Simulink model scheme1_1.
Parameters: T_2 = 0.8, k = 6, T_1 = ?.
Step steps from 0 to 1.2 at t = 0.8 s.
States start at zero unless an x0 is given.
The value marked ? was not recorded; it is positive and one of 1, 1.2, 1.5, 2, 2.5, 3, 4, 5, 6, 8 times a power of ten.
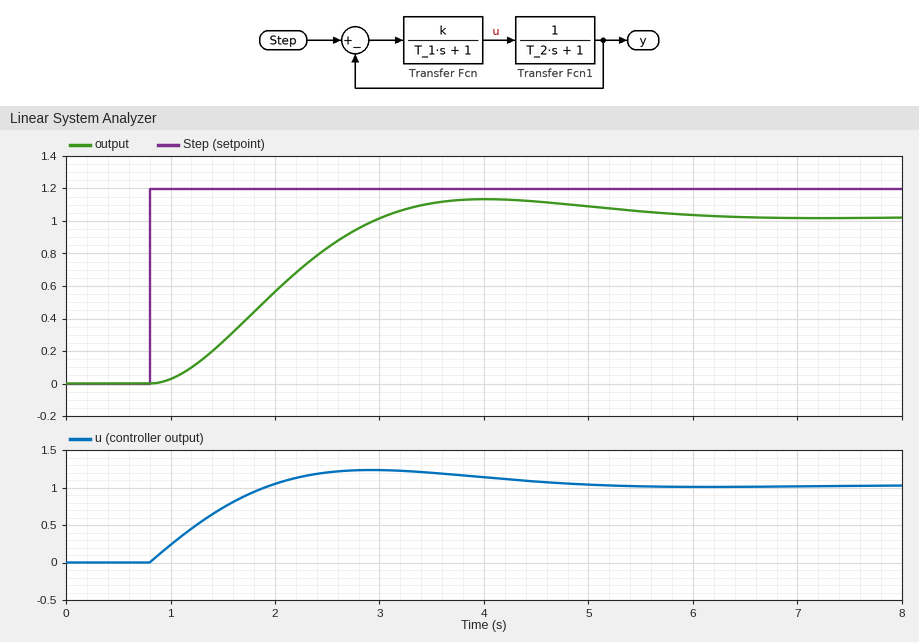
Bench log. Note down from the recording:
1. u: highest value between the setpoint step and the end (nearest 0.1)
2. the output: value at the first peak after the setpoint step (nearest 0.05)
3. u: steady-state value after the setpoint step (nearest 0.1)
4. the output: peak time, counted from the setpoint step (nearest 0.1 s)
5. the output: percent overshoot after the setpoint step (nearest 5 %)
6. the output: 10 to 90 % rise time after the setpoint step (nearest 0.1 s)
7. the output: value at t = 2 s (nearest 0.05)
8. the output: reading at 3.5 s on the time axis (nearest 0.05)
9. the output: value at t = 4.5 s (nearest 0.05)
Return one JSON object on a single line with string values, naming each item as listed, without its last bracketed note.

{"u: highest value between the setpoint step and the end": "1.2", "the output: value at the first peak after the setpoint step": "1.15", "u: steady-state value after the setpoint step": "1.0", "the output: peak time, counted from the setpoint step": "3.2 s", "the output: percent overshoot after the setpoint step": "10 %", "the output: 10 to 90 % rise time after the setpoint step": "1.5 s", "the output: value at t = 2 s": "0.55", "the output: reading at 3.5 s on the time axis": "1.10", "the output: value at t = 4.5 s": "1.10"}
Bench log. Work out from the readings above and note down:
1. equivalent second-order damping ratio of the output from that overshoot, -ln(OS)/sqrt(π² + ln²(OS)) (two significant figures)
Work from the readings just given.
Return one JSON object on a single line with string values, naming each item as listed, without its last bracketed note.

{"equivalent second-order damping ratio of the output from that overshoot, -ln(OS)/sqrt(π² + ln²(OS))": "0.59"}
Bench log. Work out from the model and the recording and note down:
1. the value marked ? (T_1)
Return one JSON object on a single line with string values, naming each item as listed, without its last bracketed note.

{"the value marked ?": "6"}
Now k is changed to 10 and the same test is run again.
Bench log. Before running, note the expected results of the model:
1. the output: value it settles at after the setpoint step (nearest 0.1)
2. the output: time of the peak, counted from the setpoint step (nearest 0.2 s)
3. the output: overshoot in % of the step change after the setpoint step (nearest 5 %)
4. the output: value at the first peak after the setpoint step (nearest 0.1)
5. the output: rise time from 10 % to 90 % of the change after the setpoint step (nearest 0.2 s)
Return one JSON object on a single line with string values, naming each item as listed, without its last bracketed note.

{"the output: value it settles at after the setpoint step": "1.1", "the output: time of the peak, counted from the setpoint step": "2.4 s", "the output: overshoot in % of the step change after the setpoint step": "20 %", "the output: value at the first peak after the setpoint step": "1.3", "the output: rise time from 10 % to 90 % of the change after the setpoint step": "1.0 s"}
